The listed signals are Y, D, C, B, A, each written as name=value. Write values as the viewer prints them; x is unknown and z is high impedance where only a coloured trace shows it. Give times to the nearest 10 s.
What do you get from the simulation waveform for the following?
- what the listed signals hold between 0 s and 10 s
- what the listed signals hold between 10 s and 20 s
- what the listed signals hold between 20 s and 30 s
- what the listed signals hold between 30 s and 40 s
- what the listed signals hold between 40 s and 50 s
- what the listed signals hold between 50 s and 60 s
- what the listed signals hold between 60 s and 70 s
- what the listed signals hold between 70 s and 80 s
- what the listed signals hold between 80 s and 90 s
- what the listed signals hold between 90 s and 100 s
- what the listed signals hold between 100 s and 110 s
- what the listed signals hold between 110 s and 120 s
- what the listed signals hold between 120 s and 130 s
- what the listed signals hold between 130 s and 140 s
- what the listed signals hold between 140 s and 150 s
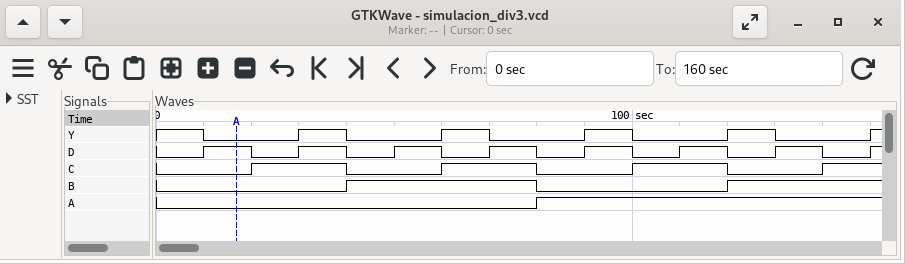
Y=1, D=0, C=0, B=0, A=0
Y=0, D=1, C=0, B=0, A=0
Y=0, D=0, C=1, B=0, A=0
Y=1, D=1, C=1, B=0, A=0
Y=0, D=0, C=0, B=1, A=0
Y=0, D=1, C=0, B=1, A=0
Y=1, D=0, C=1, B=1, A=0
Y=0, D=1, C=1, B=1, A=0
Y=0, D=0, C=0, B=0, A=1
Y=1, D=1, C=0, B=0, A=1
Y=0, D=0, C=1, B=0, A=1
Y=0, D=1, C=1, B=0, A=1
Y=1, D=0, C=0, B=1, A=1
Y=0, D=1, C=0, B=1, A=1
Y=0, D=0, C=1, B=1, A=1
